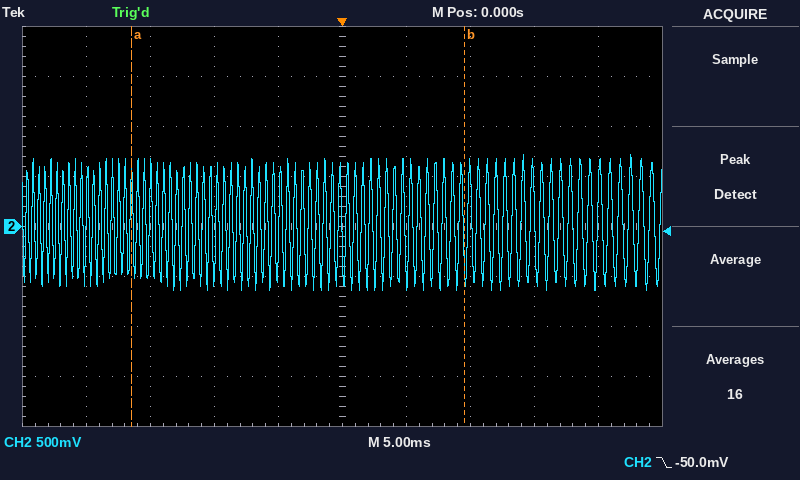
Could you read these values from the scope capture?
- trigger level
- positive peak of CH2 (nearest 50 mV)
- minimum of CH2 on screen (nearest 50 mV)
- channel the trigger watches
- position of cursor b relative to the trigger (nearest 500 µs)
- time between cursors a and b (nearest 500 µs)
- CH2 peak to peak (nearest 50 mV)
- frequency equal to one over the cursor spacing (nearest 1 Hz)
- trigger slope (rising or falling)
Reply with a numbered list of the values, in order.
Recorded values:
1. -50.0 mV
2. 700 mV
3. -650 mV
4. CH2
5. +9.5 ms
6. 26.0 ms
7. 1.35 V
8. 38 Hz
9. falling
